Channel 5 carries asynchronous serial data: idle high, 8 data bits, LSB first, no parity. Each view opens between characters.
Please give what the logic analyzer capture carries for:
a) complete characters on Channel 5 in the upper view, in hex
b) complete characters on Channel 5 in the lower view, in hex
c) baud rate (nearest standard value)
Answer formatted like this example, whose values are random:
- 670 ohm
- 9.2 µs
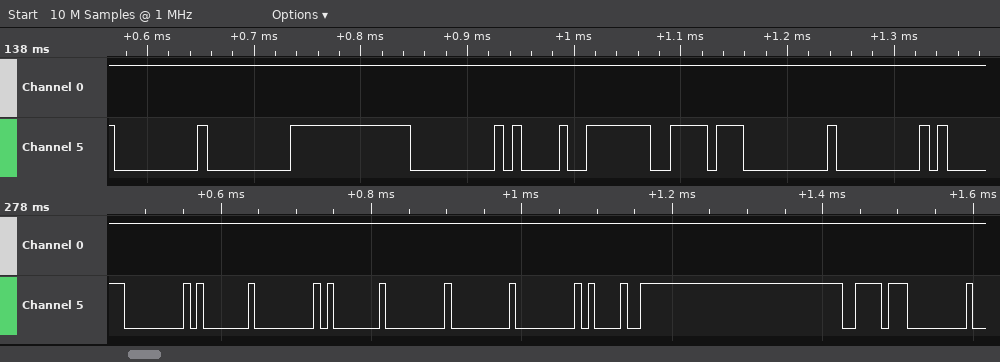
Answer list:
- 00, 00, 00, 21, DE, 00, 00
- 00, 01, 00, 01, 00, 00, 00, 21, DE, 00
- 115200 baud
